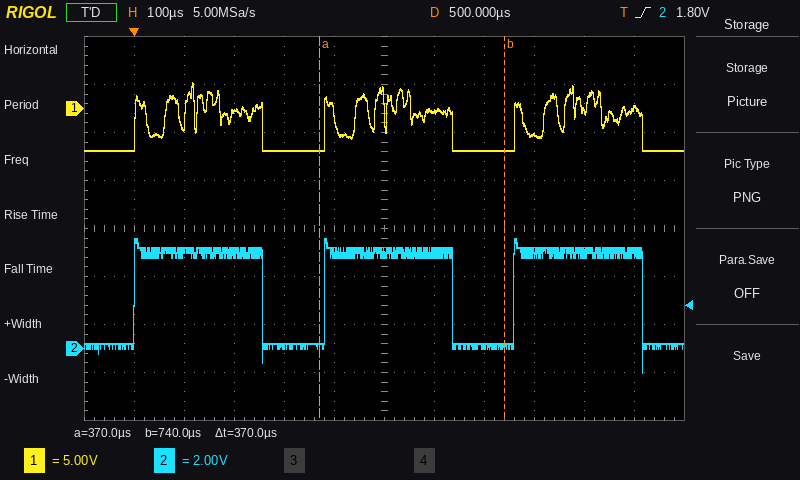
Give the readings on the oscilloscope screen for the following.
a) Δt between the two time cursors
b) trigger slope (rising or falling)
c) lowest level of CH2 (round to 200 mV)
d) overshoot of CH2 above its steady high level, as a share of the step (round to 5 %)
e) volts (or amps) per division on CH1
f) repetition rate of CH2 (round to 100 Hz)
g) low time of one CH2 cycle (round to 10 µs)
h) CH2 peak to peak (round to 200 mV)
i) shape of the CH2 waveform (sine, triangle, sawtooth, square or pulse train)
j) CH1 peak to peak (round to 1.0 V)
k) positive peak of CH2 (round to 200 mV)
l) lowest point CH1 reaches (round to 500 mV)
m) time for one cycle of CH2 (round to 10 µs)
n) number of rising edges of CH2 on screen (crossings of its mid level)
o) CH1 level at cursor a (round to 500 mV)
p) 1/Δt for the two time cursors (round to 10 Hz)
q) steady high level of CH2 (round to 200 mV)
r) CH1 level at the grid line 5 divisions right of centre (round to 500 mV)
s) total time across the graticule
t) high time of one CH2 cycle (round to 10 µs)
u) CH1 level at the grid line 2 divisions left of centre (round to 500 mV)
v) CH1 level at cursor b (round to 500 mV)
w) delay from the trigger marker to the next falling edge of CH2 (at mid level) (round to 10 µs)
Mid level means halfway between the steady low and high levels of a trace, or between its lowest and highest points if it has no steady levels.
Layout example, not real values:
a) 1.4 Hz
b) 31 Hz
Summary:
a) 370 µs
b) rising
c) -1.0 V
d) 15 %
e) 5 V
f) 2.6 kHz
g) 120 µs
h) 5.6 V
i) pulse train
j) 7.0 V
k) 4.6 V
l) -4.5 V
m) 380 µs
n) 3
o) -4.5 V
p) 2.70 kHz
q) 4.0 V
r) 0.0 V
s) 1.2 ms
t) 260 µs
u) -4.5 V
v) -4.5 V
w) 260 µs
